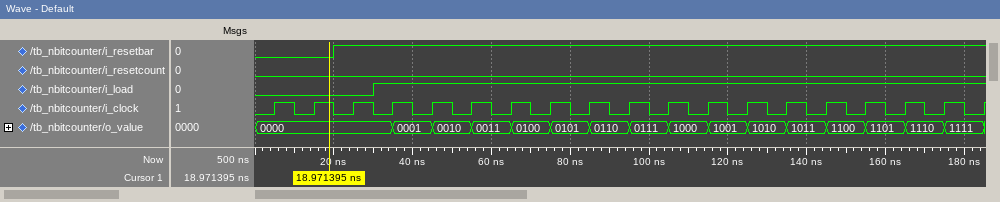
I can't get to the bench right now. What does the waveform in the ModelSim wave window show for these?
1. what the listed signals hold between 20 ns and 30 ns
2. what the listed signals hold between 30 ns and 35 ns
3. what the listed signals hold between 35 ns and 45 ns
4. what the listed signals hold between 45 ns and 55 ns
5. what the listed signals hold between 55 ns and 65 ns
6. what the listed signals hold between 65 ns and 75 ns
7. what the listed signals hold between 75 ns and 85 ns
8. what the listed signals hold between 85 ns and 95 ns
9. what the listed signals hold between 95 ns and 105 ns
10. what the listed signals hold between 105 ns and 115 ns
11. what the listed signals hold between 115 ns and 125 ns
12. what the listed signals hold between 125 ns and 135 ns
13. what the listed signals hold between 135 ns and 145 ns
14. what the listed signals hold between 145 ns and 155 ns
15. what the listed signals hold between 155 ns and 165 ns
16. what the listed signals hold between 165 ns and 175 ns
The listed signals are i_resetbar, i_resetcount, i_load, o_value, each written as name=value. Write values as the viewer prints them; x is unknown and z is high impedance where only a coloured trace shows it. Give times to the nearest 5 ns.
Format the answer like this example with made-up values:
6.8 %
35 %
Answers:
i_resetbar=1, i_resetcount=0, i_load=0, o_value=0000
i_resetbar=1, i_resetcount=0, i_load=1, o_value=0000
i_resetbar=1, i_resetcount=0, i_load=1, o_value=0001
i_resetbar=1, i_resetcount=0, i_load=1, o_value=0010
i_resetbar=1, i_resetcount=0, i_load=1, o_value=0011
i_resetbar=1, i_resetcount=0, i_load=1, o_value=0100
i_resetbar=1, i_resetcount=0, i_load=1, o_value=0101
i_resetbar=1, i_resetcount=0, i_load=1, o_value=0110
i_resetbar=1, i_resetcount=0, i_load=1, o_value=0111
i_resetbar=1, i_resetcount=0, i_load=1, o_value=1000
i_resetbar=1, i_resetcount=0, i_load=1, o_value=1001
i_resetbar=1, i_resetcount=0, i_load=1, o_value=1010
i_resetbar=1, i_resetcount=0, i_load=1, o_value=1011
i_resetbar=1, i_resetcount=0, i_load=1, o_value=1100
i_resetbar=1, i_resetcount=0, i_load=1, o_value=1101
i_resetbar=1, i_resetcount=0, i_load=1, o_value=1110
